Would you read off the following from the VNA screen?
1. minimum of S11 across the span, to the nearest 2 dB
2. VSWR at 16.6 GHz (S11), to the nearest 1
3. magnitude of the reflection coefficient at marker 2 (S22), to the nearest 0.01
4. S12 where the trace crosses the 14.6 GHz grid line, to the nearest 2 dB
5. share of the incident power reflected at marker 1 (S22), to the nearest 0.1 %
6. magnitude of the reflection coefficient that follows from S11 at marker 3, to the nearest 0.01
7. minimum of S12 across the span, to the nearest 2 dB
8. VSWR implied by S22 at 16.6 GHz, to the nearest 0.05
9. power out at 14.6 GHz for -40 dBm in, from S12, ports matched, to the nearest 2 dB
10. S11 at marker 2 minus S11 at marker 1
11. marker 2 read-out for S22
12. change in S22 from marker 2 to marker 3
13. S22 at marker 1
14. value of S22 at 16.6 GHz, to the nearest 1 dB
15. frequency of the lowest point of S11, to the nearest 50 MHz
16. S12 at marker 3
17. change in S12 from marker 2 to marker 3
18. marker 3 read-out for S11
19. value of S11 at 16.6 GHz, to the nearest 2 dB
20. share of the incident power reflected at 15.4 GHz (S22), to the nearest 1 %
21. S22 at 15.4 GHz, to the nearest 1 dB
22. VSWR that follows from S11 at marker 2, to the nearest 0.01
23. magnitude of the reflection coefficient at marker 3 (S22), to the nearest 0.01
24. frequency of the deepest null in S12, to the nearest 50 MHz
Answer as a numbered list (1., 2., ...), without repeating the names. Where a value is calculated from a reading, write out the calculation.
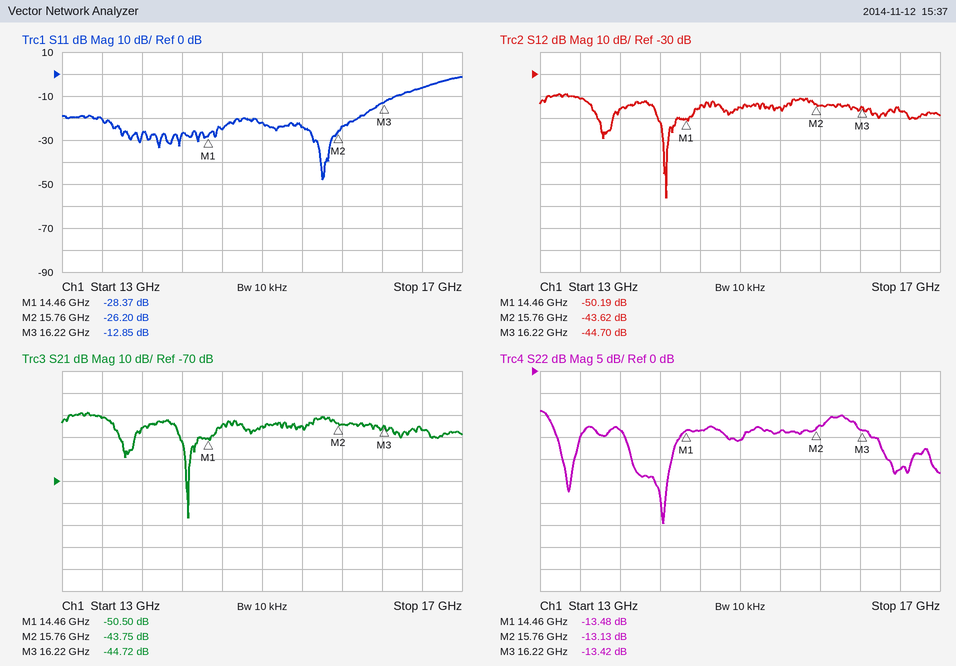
1. -48 dB
2. |Γ| = 10^(-6/20) = 0.5012; VSWR = (1 + 0.5012)/(1 − 0.5012) ≈ 3
3. 10^(-13.13/20) ≈ 0.22
4. -44 dB
5. 10^(-13.48/10) ≈ 4.5 %
6. 10^(-12.85/20) ≈ 0.23
7. -86 dB
8. |Γ| = 10^(-22/20) = 0.0794; VSWR = (1 + 0.0794)/(1 − 0.0794) ≈ 1.17, so 1.15 to the nearest 0.05
9. -40 dBm + (-44 dB) = -84 dBm
10. -26.2 − (-28.37) = 2.17 dB
11. -13.13 dB
12. -13.42 − (-13.13) = -0.29 dB
13. -13.48 dB
14. -22 dB
15. 15.60 GHz
16. -44.70 dB
17. -44.7 − (-43.62) = -1.08 dB
18. -12.85 dB
19. -6 dB
20. 10^(-14/10) ≈ 4 %
21. -14 dB
22. (1 + 0.0490)/(1 − 0.0490) ≈ 1.10
23. 10^(-13.42/20) ≈ 0.21
24. 14.25 GHz
